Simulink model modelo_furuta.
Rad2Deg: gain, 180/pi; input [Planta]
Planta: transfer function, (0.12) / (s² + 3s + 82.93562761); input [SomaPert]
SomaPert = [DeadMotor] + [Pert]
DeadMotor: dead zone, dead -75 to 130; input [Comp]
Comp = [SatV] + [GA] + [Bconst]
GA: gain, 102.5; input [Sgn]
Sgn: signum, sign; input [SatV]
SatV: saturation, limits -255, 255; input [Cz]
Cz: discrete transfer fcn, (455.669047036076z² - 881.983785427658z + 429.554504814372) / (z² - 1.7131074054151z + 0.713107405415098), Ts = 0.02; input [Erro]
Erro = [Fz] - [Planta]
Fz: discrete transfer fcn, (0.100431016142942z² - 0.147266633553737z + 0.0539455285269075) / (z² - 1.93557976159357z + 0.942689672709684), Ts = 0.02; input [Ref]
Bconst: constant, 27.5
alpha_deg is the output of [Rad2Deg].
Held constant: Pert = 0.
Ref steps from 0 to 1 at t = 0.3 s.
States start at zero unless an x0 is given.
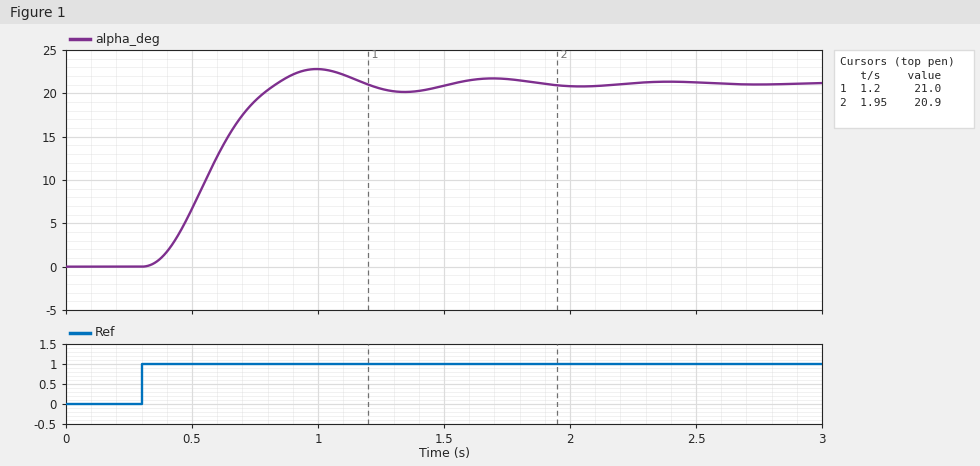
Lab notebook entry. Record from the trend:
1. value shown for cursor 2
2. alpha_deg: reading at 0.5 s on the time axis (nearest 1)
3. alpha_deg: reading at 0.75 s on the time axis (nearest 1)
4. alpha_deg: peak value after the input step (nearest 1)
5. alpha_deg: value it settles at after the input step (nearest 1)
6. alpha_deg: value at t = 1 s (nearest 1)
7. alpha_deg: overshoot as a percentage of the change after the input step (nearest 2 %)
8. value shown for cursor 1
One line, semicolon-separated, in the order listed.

20.9; 7; 19; 23; 21; 23; 8 %; 21.0
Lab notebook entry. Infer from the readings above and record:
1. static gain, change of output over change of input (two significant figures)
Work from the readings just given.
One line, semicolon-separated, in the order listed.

21
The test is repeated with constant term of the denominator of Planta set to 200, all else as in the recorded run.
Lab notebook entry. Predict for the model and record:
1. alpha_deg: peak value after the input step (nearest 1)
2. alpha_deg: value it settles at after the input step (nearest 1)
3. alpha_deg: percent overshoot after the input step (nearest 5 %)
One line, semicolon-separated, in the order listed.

10; 9; 10 %
